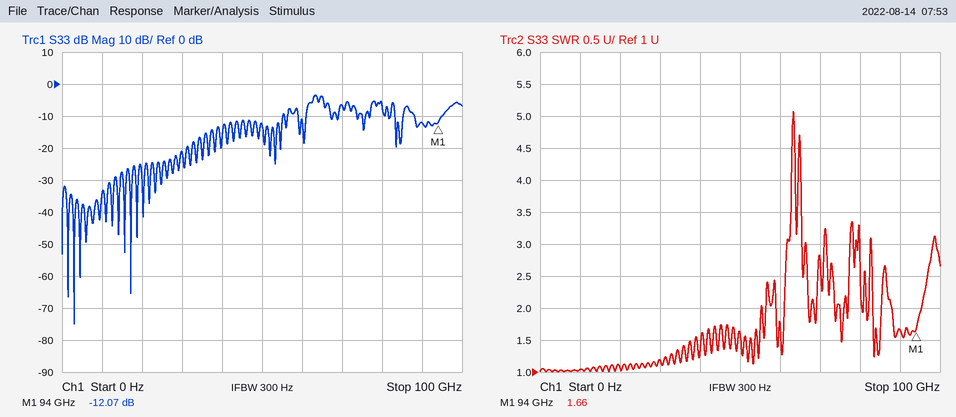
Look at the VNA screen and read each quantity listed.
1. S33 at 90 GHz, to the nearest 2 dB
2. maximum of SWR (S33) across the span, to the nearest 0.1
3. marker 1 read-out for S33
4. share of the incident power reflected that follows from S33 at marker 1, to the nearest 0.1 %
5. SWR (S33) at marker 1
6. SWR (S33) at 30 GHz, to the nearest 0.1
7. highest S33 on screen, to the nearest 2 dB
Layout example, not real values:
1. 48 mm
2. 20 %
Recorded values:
1. -12 dB
2. 5.1
3. -12.07 dB
4. 6.2 %
5. 1.66
6. 1.2
7. -4 dB
